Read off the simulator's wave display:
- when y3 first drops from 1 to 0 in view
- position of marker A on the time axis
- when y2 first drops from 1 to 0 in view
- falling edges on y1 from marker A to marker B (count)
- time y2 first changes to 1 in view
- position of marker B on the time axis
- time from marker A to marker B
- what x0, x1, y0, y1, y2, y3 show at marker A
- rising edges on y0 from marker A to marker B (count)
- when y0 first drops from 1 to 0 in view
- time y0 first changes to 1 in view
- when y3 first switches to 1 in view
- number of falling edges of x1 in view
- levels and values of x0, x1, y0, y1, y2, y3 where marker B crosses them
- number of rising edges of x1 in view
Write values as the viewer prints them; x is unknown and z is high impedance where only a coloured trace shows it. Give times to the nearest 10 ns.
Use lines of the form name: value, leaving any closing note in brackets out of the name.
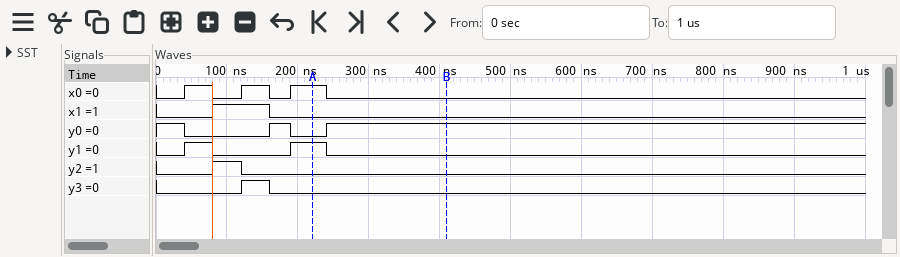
when y3 first drops from 1 to 0 in view: 160 ns
position of marker A on the time axis: 220 ns
when y2 first drops from 1 to 0 in view: 120 ns
falling edges on y1 from marker A to marker B: 1
time y2 first changes to 1 in view: 80 ns
position of marker B on the time axis: 410 ns
time from marker A to marker B: 190 ns
what x0, x1, y0, y1, y2, y3 show at marker A: x0=1, x1=0, y0=0, y1=1, y2=0, y3=0
rising edges on y0 from marker A to marker B: 1
when y0 first drops from 1 to 0 in view: 40 ns
time y0 first changes to 1 in view: 160 ns
when y3 first switches to 1 in view: 120 ns
number of falling edges of x1 in view: 1
levels and values of x0, x1, y0, y1, y2, y3 where marker B crosses them: x0=0, x1=0, y0=1, y1=0, y2=0, y3=0
number of rising edges of x1 in view: 1
